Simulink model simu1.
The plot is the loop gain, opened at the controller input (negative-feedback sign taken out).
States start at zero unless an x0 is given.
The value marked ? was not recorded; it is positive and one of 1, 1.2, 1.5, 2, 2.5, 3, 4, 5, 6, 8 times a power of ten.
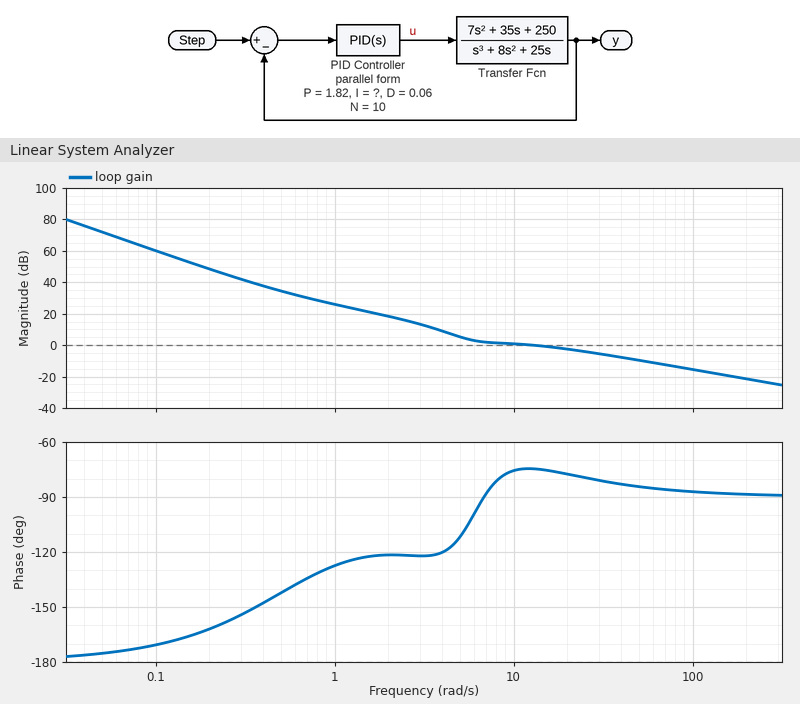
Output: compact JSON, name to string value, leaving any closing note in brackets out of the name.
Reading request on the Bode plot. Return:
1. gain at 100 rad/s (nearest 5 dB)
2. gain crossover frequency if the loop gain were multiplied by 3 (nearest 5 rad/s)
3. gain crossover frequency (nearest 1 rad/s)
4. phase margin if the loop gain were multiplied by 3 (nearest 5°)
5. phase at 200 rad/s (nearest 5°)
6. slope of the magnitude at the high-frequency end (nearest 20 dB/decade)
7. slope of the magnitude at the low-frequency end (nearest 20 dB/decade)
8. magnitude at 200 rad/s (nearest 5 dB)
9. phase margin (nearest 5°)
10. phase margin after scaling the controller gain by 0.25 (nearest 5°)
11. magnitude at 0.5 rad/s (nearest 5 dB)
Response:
{"gain at 100 rad/s": "-15 dB", "gain crossover frequency if the loop gain were multiplied by 3": "50 rad/s", "gain crossover frequency": "13 rad/s", "phase margin if the loop gain were multiplied by 3": "95°", "phase at 200 rad/s": "-90°", "slope of the magnitude at the high-frequency end": "-20 dB/decade", "slope of the magnitude at the low-frequency end": "-40 dB/decade", "magnitude at 200 rad/s": "-20 dB", "phase margin": "105°", "phase margin after scaling the controller gain by 0.25": "60°", "magnitude at 0.5 rad/s": "35 dB"}
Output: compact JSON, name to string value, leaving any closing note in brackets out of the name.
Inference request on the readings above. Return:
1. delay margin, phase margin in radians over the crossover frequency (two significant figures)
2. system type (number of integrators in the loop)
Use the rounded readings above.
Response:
{"delay margin, phase margin in radians over the crossover frequency": "0.14 s", "system type": "2"}
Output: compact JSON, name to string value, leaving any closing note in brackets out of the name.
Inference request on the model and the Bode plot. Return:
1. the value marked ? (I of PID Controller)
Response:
{"the value marked ?": "1"}
